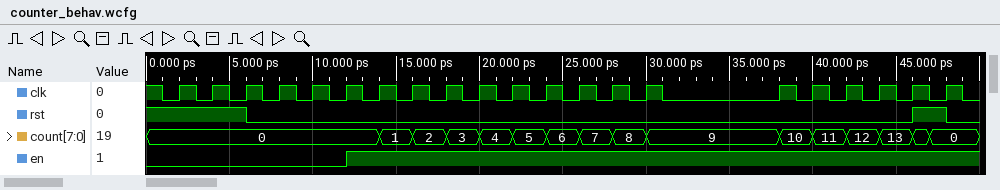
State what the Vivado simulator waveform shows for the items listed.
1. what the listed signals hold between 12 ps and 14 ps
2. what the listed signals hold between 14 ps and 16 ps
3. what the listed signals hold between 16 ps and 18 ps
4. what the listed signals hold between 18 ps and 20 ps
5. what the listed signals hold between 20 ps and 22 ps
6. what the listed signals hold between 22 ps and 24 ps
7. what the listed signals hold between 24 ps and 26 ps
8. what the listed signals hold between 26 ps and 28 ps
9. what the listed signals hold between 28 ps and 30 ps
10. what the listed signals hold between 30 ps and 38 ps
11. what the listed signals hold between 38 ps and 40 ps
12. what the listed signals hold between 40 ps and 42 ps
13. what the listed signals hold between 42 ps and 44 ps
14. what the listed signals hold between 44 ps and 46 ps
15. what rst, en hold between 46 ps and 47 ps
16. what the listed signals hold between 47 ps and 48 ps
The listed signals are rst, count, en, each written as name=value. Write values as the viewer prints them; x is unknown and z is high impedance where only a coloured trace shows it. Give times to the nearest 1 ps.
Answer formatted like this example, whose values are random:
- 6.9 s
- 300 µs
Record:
- rst=0, count=0, en=1
- rst=0, count=1, en=1
- rst=0, count=2, en=1
- rst=0, count=3, en=1
- rst=0, count=4, en=1
- rst=0, count=5, en=1
- rst=0, count=6, en=1
- rst=0, count=7, en=1
- rst=0, count=8, en=1
- rst=0, count=9, en=1
- rst=0, count=10, en=1
- rst=0, count=11, en=1
- rst=0, count=12, en=1
- rst=0, count=13, en=1
- rst=1, en=1
- rst=1, count=0, en=1
